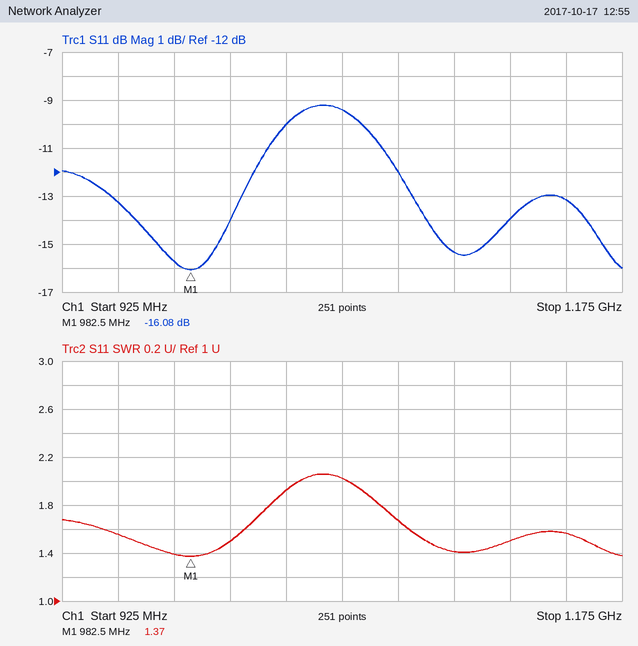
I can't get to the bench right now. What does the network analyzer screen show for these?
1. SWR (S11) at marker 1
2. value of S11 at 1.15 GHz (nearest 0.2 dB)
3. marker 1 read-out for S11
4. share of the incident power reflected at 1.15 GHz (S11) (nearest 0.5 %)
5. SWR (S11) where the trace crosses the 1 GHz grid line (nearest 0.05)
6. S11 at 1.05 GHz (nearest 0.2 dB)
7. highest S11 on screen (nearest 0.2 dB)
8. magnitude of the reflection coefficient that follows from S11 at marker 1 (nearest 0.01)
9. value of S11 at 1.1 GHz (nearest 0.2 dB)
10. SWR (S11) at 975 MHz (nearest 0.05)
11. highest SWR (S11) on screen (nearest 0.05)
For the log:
1.37
-13.2 dB
-16.08 dB
5.0 %
1.50
-9.4 dB
-9.2 dB
0.16
-15.4 dB
1.40
2.05
